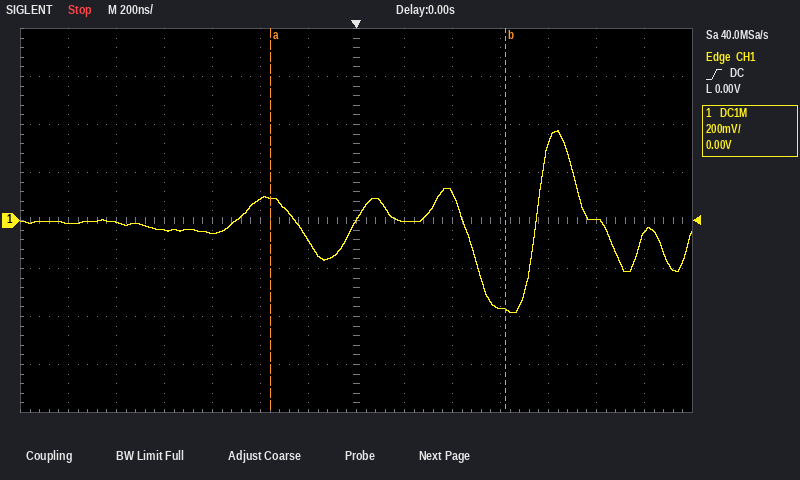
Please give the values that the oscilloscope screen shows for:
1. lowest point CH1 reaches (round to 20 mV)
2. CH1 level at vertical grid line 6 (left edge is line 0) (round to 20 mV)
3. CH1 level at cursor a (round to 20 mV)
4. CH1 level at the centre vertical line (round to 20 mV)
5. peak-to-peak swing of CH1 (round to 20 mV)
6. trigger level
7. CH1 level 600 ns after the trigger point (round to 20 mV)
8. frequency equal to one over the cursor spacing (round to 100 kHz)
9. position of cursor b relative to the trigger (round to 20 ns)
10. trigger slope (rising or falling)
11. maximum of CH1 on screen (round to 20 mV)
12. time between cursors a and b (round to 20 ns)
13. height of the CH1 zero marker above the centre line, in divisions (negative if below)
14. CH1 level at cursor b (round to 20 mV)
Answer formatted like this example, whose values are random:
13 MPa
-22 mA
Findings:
-380 mV
-80 mV
100 mV
0 mV
760 mV
0.00 V
-360 mV
1.0 MHz
+620 ns
rising
380 mV
980 ns
0.0 div
-380 mV
